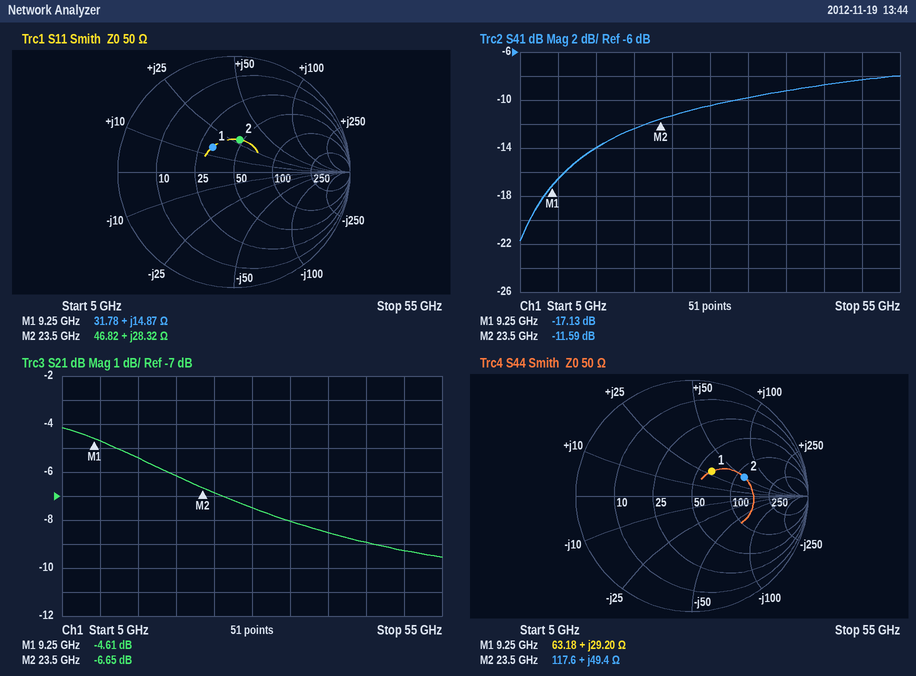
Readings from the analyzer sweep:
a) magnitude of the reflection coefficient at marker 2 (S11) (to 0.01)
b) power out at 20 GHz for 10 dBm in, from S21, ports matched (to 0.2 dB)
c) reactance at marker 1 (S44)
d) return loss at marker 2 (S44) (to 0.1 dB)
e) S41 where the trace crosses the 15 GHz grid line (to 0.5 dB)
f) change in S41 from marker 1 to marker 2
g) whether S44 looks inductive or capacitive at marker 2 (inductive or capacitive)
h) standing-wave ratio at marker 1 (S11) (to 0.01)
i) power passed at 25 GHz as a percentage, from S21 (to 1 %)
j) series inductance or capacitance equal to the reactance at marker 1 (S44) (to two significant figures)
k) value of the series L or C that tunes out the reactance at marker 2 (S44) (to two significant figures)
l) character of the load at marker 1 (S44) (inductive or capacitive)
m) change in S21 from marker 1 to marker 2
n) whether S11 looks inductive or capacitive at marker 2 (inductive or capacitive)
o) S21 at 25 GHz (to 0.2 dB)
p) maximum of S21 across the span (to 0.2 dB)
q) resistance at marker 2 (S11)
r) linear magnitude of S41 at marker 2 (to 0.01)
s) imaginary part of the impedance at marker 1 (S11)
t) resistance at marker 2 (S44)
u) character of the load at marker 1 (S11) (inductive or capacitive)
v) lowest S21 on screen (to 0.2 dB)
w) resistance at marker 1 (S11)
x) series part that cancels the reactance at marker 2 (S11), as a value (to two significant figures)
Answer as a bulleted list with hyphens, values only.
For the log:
- 0.28
- 3.8 dBm
- +29.20 Ω
- 6.4 dB
- -14.0 dB
- 5.54 dB
- inductive
- 1.79
- 21 %
- 500 pH
- 140 fF
- inductive
- -2.04 dB
- inductive
- -6.8 dB
- -4.2 dB
- 46.82 Ω
- 0.26
- +14.87 Ω
- 117.6 Ω
- inductive
- -9.6 dB
- 31.78 Ω
- 240 fF
